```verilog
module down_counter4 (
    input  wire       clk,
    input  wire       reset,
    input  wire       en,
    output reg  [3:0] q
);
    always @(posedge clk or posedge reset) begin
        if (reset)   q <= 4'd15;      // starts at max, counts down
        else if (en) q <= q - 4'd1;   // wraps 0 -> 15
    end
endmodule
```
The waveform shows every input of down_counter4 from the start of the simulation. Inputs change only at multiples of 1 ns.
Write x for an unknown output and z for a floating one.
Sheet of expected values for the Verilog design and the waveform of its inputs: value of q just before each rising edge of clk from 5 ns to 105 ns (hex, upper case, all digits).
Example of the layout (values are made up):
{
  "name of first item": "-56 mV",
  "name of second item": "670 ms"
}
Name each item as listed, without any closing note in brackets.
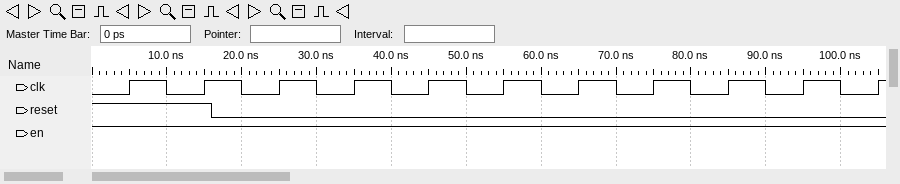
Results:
{
  "value of q just before each rising edge of clk from 5 ns to 105 ns": "F, F, F, E, D, C, B, A, 9, 8, 7"
}
